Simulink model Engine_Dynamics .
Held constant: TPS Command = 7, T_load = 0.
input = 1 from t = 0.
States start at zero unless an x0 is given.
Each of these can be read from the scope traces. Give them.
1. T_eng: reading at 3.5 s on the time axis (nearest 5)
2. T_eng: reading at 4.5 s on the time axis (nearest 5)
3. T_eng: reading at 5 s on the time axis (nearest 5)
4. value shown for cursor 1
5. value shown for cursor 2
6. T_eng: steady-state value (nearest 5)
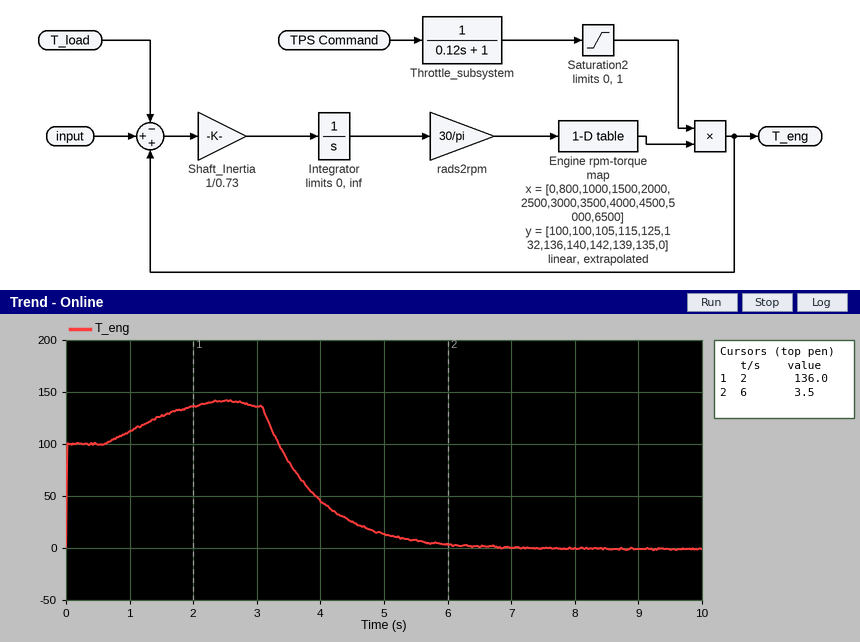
85
25
15
136.0
3.5
0
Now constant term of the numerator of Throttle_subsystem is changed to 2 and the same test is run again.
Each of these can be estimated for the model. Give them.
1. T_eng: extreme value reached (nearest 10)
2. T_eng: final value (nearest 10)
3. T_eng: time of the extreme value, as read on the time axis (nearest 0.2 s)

140
0
2.6 s
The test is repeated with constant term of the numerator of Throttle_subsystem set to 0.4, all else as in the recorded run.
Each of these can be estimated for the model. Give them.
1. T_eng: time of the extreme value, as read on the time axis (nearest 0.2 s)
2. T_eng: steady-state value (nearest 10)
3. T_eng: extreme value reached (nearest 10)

2.6 s
0
140
